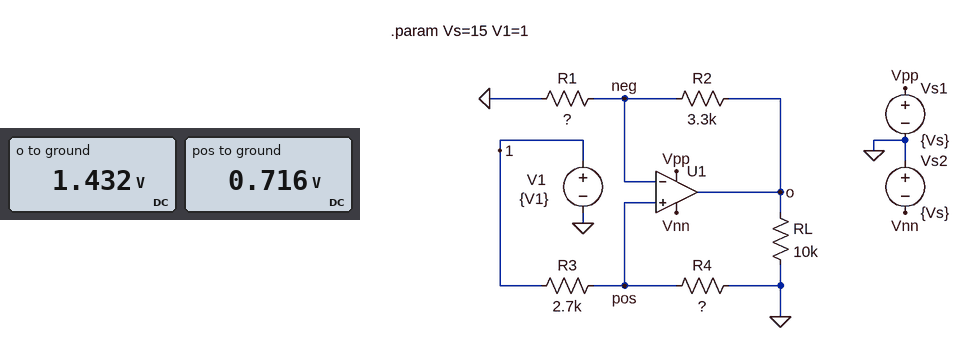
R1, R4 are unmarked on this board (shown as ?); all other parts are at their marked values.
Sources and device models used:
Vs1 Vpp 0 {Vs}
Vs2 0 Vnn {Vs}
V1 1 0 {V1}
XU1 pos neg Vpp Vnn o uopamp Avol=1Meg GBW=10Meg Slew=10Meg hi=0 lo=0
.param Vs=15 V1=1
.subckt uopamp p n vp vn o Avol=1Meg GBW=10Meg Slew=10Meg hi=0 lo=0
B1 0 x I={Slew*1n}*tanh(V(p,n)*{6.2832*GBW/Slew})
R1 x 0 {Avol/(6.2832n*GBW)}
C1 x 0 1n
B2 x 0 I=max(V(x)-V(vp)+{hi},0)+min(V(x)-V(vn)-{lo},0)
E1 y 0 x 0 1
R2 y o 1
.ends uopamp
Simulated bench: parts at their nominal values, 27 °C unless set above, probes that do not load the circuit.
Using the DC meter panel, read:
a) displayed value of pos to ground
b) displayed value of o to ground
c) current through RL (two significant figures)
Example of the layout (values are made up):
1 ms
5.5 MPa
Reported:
0.716 V
1.432 V
140 µA
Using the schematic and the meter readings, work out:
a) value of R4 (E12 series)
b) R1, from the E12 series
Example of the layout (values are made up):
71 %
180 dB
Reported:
6.8 kΩ
3.3 kΩ
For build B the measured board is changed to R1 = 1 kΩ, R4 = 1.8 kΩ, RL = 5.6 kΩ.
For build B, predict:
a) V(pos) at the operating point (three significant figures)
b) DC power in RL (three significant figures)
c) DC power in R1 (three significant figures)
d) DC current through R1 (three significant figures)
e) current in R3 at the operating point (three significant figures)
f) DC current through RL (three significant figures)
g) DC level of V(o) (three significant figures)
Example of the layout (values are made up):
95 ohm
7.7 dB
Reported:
400 mV
528 µW
160 µW
400 µA
222 µA
307 µA
1.72 V
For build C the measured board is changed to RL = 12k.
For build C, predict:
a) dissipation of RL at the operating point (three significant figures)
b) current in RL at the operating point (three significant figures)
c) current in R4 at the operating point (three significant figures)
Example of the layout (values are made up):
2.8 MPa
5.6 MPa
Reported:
171 µW
119 µA
105 µA
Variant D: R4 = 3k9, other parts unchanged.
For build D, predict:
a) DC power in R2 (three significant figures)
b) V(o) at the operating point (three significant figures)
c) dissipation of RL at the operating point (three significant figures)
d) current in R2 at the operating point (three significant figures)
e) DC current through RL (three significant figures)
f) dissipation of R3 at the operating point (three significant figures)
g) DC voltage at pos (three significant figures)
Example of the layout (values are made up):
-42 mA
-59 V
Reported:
106 µW
1.18 V
140 µW
179 µA
118 µA
62.0 µW
591 mV
